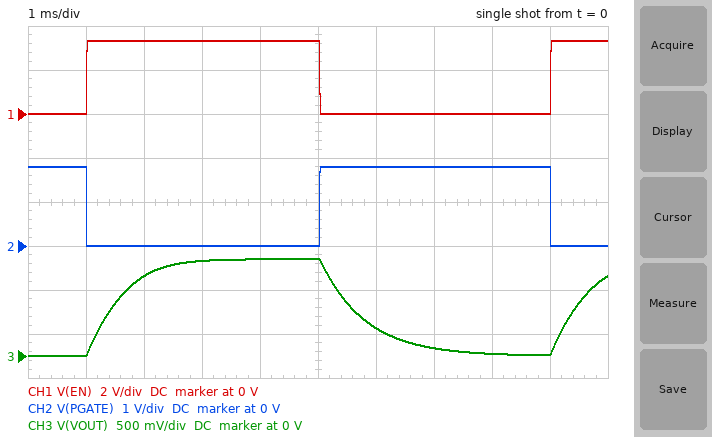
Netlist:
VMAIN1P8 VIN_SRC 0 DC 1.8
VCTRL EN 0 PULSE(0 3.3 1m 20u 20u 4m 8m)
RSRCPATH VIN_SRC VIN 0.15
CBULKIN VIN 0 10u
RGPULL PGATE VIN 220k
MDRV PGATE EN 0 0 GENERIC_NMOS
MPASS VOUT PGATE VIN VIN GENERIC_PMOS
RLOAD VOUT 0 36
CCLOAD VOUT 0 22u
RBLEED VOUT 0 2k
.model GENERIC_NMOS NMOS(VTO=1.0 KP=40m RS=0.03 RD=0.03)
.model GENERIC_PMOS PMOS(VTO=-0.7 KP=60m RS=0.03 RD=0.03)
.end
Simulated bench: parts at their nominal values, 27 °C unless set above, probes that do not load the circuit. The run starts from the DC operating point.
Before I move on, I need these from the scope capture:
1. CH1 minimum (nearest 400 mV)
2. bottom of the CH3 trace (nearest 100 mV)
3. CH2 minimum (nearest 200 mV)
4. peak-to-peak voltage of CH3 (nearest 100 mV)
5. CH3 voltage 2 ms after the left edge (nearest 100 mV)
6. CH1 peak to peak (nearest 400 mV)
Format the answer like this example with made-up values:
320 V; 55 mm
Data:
0 V; 0 V; 0 V; 1.1 V; 900 mV; 3.2 V
